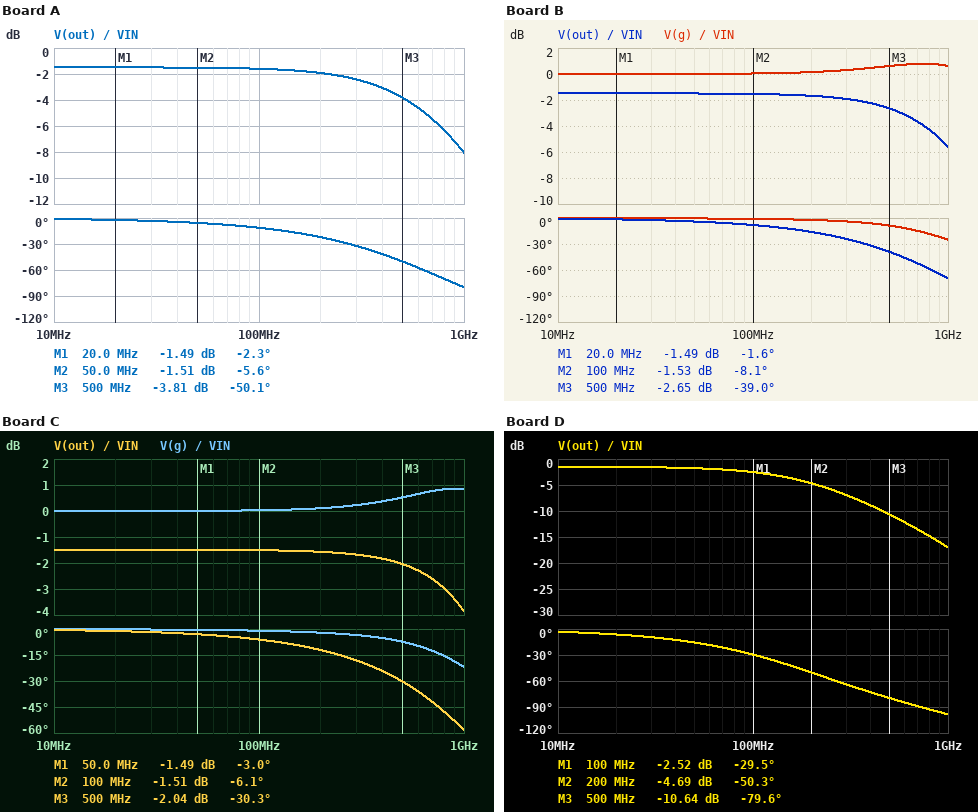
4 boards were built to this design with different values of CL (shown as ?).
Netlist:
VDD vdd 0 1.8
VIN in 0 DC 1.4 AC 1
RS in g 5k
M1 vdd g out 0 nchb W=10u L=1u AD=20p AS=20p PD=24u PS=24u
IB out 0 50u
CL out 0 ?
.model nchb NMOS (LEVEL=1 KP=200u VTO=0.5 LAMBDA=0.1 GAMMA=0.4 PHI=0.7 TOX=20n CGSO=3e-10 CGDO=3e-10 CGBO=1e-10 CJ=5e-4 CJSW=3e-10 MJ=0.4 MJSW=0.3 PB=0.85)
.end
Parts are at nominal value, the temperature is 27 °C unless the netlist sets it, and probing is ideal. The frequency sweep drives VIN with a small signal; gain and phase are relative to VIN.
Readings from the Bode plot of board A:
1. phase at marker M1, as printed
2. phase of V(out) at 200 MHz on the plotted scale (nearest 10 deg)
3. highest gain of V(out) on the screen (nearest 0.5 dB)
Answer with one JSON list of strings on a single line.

["-2.3 deg", "-20 deg", "-1.5 dB"]
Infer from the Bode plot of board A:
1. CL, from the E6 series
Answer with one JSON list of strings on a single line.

["150 fF"]
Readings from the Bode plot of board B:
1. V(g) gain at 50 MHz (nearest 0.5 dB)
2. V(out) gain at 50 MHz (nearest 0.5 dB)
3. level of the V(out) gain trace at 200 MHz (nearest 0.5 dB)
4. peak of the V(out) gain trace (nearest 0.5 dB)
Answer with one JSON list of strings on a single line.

["0 dB", "-1.5 dB", "-1.5 dB", "-1.5 dB"]
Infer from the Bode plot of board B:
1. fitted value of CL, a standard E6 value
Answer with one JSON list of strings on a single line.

["100 fF"]
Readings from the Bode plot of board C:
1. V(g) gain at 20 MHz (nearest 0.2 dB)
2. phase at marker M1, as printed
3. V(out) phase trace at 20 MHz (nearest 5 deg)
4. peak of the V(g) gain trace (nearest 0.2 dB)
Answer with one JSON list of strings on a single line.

["0 dB", "-3.0 deg", "0 deg", "0.8 dB"]
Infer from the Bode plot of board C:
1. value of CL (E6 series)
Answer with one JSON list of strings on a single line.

["68 fF"]
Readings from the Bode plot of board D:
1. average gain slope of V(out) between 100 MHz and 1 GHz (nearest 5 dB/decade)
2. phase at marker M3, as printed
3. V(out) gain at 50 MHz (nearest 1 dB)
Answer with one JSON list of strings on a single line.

["-15 dB/decade", "-79.6 deg", "-2 dB"]
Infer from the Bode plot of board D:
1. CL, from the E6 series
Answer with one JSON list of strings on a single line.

["470 fF"]
